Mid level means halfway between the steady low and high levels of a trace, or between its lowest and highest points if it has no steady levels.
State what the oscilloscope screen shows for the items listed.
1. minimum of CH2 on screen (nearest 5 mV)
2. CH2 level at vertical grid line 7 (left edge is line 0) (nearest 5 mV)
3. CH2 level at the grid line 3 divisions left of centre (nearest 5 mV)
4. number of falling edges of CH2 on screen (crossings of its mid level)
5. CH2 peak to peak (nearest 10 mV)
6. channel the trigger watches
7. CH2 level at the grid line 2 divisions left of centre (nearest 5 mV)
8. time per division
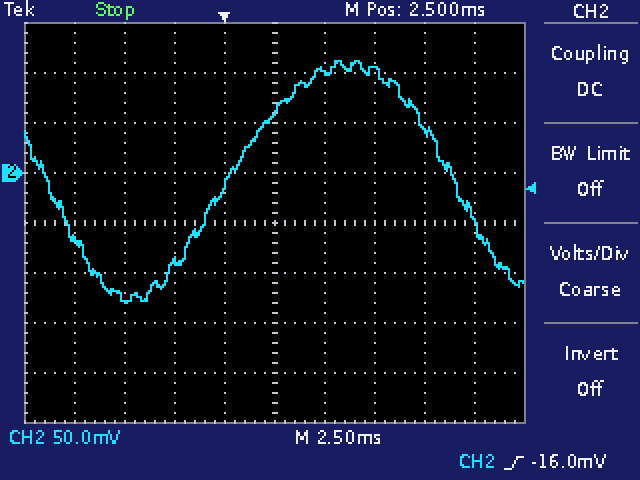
-130 mV
105 mV
-125 mV
2
240 mV
CH2
-90 mV
2.5 ms
